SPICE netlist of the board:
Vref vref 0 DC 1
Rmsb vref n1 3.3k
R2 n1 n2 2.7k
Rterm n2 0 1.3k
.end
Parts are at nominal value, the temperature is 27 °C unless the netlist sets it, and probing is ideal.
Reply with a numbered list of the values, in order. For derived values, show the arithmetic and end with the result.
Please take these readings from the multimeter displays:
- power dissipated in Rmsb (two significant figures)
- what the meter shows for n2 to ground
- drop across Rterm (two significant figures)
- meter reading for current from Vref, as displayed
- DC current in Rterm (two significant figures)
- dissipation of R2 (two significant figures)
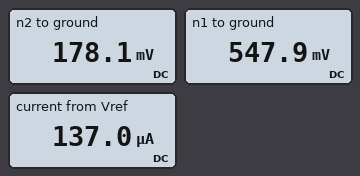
1. (1 V - 547.9 mV)^2 / 3.3 kΩ = 62 µW
2. 178.1 mV
3. 178.1 mV = 180 mV
4. 137.0 µA
5. (178.1 mV) / 1.3 kΩ = 140 µA
6. (547.9 mV - 178.1 mV)^2 / 2.7 kΩ = 51 µW
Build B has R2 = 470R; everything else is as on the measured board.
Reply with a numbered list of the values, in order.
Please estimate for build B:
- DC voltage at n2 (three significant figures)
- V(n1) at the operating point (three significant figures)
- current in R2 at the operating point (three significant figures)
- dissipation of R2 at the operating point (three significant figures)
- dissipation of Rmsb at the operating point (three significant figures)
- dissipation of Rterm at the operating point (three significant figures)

1. 256 mV
2. 349 mV
3. 197 µA
4. 18.3 µW
5. 128 µW
6. 50.6 µW
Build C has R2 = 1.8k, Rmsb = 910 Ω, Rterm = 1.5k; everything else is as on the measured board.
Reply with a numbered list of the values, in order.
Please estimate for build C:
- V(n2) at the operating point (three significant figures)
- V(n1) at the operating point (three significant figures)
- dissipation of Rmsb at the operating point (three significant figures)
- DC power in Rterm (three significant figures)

1. 356 mV
2. 784 mV
3. 51.3 µW
4. 84.6 µW
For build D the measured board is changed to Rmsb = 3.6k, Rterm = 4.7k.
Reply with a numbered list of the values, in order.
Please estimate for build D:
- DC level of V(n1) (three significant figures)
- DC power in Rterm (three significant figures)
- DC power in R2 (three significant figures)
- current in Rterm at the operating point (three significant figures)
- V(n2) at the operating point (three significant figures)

1. 673 mV
2. 38.8 µW
3. 22.3 µW
4. 90.9 µA
5. 427 mV
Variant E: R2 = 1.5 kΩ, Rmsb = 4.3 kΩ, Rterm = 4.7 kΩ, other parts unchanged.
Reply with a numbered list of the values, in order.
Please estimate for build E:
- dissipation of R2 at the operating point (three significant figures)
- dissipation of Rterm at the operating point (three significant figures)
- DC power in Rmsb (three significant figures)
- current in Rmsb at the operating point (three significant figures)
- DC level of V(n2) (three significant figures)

1. 13.6 µW
2. 42.6 µW
3. 39.0 µW
4. 95.2 µA
5. 448 mV
